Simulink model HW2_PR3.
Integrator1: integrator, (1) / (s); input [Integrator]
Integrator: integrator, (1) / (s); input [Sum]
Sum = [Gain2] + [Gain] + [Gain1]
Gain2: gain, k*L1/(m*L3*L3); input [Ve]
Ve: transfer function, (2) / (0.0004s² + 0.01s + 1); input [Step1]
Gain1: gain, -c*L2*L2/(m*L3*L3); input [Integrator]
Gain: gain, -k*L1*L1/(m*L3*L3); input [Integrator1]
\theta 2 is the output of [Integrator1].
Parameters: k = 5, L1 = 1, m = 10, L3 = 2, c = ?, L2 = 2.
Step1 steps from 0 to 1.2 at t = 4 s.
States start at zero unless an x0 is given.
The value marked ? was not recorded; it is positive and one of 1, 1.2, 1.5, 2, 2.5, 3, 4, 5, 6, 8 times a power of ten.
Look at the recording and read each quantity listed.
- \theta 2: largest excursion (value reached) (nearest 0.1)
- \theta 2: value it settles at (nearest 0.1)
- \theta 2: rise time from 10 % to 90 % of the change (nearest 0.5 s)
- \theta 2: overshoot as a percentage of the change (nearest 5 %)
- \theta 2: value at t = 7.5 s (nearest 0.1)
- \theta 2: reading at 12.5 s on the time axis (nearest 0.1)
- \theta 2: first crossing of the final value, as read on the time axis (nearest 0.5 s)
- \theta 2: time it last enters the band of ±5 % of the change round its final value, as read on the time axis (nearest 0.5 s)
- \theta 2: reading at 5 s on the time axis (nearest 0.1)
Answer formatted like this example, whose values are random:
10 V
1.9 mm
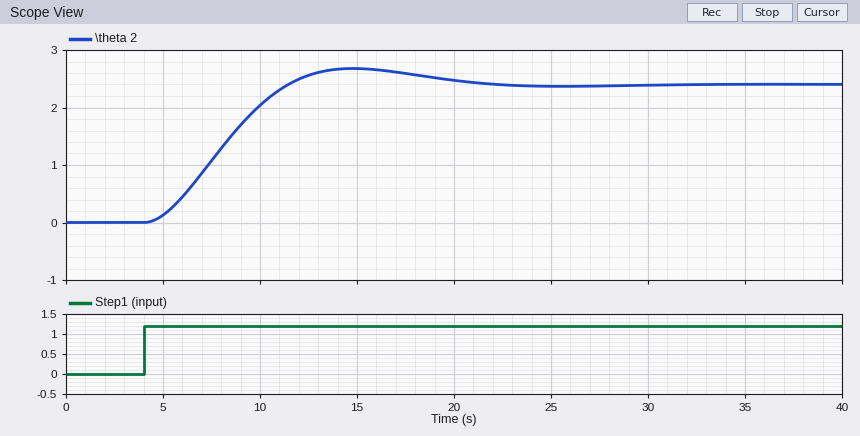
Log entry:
2.7
2.4
5.0 s
10 %
1.1
2.6
11.5 s
19.0 s
0.1
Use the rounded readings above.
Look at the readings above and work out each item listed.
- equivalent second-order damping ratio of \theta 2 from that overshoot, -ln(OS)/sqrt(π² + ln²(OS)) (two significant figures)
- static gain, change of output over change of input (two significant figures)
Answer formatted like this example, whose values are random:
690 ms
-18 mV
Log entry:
0.59
2.0
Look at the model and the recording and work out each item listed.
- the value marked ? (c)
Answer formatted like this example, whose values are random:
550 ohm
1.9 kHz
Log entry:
4
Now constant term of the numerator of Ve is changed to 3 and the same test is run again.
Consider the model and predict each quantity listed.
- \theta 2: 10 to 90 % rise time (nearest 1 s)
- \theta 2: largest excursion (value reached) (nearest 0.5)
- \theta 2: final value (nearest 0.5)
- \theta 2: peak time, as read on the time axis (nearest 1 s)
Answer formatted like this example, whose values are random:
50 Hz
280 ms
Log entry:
5 s
4.0
3.5
15 s
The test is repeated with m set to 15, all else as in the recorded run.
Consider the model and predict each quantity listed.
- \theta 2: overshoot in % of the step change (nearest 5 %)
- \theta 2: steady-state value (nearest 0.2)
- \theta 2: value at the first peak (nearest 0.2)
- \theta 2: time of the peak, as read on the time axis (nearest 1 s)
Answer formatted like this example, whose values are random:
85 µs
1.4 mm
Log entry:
20 %
2.4
2.8
16 s
